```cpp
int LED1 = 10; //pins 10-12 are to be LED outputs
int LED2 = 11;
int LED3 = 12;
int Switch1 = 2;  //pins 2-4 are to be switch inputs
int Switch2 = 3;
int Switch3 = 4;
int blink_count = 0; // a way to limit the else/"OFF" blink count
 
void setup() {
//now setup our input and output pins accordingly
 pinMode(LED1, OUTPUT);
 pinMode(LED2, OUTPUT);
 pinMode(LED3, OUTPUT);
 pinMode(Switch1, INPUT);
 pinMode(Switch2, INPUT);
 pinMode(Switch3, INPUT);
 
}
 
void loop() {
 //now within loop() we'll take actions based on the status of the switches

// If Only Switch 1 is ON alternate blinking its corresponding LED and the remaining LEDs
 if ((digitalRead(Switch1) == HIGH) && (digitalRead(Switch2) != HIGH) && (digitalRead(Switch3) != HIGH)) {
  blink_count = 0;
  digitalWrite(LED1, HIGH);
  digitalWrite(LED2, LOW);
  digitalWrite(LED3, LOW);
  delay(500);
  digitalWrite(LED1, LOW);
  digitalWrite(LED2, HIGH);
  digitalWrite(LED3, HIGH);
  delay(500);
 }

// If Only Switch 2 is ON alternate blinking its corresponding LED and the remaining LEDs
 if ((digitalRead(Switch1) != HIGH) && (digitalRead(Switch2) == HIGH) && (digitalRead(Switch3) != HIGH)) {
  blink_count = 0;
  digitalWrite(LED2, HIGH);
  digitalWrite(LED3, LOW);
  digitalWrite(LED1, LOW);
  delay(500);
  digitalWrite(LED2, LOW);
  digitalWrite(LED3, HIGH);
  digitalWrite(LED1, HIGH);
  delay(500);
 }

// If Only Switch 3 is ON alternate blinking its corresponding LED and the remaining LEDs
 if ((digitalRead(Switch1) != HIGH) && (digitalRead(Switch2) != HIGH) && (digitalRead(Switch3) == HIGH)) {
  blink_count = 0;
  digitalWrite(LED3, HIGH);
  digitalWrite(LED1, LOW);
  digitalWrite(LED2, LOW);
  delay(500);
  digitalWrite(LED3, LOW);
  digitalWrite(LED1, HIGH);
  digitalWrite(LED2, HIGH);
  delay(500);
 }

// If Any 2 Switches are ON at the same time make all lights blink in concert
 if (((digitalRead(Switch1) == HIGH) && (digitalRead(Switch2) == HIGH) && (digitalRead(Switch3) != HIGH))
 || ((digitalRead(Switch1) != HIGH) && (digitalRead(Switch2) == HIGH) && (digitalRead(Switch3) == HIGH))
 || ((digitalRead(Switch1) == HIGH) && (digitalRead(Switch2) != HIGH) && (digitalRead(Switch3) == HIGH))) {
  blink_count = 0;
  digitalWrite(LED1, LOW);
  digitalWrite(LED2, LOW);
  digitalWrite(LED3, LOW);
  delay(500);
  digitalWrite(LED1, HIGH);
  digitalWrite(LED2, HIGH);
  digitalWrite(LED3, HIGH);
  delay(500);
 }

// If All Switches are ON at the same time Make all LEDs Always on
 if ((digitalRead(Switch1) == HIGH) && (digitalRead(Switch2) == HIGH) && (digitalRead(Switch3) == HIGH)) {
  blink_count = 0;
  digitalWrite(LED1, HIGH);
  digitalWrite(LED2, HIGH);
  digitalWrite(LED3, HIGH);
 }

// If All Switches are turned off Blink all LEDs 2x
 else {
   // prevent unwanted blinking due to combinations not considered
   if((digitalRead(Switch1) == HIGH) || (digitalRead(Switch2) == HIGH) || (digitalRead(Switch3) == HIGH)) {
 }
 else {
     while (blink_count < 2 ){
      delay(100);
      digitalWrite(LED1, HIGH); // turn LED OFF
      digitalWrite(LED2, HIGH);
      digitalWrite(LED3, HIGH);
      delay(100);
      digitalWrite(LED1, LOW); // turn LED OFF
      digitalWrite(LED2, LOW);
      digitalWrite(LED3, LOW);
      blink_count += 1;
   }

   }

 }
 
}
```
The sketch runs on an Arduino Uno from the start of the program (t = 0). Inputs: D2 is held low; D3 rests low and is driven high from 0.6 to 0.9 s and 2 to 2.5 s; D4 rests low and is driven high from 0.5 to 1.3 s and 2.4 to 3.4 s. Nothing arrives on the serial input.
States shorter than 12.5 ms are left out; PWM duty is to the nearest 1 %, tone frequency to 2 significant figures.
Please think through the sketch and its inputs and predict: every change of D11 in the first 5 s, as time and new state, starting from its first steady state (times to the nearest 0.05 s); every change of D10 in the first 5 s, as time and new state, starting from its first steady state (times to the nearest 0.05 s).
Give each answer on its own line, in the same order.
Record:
0 s low; 0.1 s high; 0.2 s low; 0.3 s high; 0.4 s low; 1 s high; 1.7 s low; 1.8 s high; 1.9 s low; 2 s high; 2.5 s low; 3.5 s high; 4.2 s low; 4.3 s high; 4.4 s low
0 s low; 0.1 s high; 0.2 s low; 0.3 s high; 0.4 s low; 1 s high; 1.7 s low; 1.8 s high; 1.9 s low; 2.5 s high; 3 s low; 3.5 s high; 4.2 s low; 4.3 s high; 4.4 s low
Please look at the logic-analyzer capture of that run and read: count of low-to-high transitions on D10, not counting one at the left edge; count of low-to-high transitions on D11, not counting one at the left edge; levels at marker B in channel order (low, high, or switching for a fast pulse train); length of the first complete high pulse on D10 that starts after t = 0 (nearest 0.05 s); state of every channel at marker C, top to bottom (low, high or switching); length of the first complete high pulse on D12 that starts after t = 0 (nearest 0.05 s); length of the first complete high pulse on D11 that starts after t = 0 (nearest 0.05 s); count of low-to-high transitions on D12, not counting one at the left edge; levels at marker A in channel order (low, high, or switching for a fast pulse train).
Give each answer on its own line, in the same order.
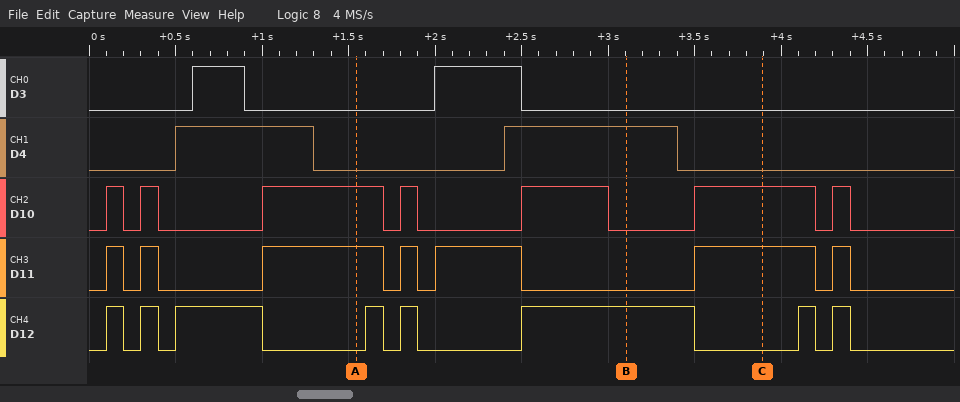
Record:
7
7
D3 low, D4 high, D10 low, D11 low, D12 high
0.10 s
D3 low, D4 low, D10 high, D11 high, D12 low
0.10 s
0.10 s
8
D3 low, D4 low, D10 high, D11 high, D12 low
